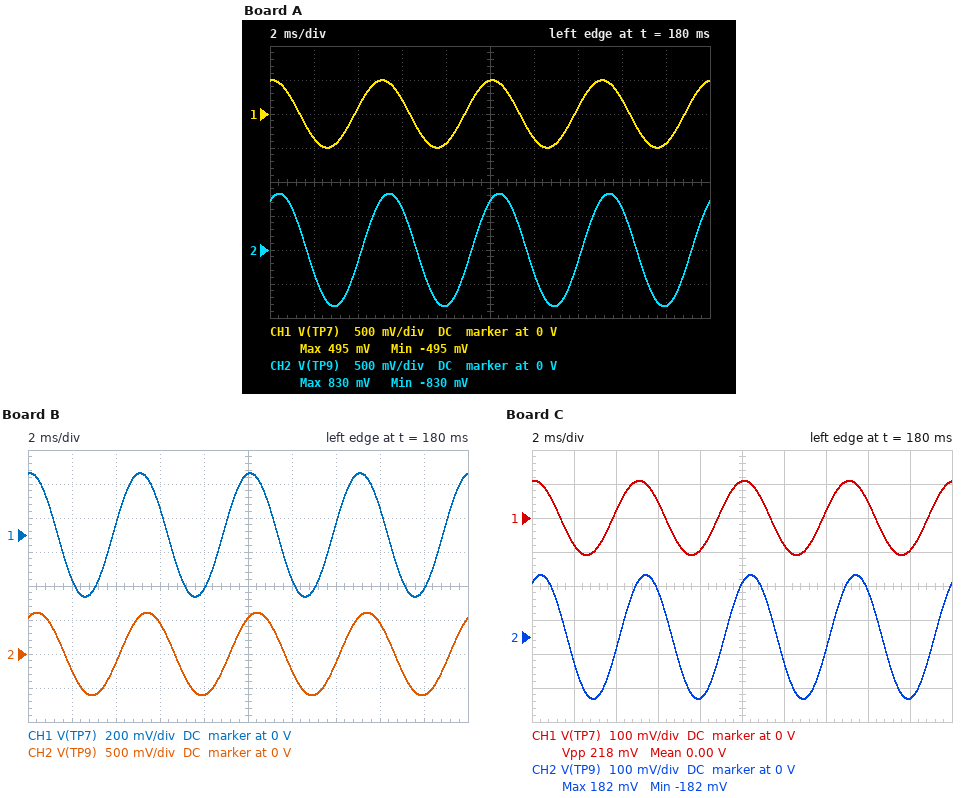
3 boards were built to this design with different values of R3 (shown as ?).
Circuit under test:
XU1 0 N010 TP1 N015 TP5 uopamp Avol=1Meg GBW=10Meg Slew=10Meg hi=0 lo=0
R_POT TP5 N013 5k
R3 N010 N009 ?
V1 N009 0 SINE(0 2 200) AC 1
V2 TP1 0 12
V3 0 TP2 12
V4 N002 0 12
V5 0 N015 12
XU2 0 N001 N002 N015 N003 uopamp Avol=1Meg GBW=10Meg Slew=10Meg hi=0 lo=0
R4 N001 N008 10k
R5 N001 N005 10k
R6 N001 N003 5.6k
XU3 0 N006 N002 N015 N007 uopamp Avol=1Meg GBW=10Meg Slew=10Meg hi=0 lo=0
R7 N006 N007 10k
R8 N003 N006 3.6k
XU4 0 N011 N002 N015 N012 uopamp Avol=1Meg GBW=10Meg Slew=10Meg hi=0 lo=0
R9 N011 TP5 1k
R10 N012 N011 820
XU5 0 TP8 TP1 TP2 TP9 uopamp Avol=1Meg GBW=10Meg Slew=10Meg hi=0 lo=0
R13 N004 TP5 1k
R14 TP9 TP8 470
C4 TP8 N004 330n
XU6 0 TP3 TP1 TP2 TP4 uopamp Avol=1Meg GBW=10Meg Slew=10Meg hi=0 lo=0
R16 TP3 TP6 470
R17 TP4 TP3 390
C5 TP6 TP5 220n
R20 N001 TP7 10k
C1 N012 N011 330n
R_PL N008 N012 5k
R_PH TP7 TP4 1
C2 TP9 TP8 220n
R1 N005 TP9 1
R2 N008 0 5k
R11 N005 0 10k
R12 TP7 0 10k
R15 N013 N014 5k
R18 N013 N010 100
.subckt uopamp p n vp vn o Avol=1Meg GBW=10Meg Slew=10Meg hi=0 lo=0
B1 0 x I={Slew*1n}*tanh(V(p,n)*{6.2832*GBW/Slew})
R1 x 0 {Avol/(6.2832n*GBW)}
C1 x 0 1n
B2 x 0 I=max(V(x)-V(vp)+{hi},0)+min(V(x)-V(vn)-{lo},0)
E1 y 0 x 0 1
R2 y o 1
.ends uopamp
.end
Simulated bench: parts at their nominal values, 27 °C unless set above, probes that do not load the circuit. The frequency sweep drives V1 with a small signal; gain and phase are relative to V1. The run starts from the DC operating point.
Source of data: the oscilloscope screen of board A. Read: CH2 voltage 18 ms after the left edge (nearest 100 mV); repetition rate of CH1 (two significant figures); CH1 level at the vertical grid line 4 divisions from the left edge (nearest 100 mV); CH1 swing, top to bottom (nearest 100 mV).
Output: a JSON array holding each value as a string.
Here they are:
["-800 mV", "200 Hz", "-400 mV", "1.0 V"]
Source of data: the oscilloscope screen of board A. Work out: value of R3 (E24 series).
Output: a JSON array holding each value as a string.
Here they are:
["2.2 kΩ"]
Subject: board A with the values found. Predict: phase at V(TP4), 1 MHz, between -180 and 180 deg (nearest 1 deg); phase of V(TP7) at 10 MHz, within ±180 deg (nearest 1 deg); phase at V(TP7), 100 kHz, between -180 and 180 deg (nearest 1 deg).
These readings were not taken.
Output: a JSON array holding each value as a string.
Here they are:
["-29 deg", "-135 deg", "-2 deg"]
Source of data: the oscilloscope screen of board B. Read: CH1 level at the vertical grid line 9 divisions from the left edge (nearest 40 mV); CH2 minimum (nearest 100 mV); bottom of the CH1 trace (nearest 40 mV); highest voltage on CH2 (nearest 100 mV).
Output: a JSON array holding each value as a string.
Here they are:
["-320 mV", "-600 mV", "-360 mV", "600 mV"]
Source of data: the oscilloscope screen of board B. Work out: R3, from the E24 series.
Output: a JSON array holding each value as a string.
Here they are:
["3 kΩ"]
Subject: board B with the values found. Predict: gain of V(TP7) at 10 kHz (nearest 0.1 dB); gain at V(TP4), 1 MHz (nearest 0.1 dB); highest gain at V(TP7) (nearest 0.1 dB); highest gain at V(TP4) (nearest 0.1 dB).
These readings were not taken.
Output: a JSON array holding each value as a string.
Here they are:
["2.9 dB", "2.5 dB", "3.0 dB", "3.0 dB"]
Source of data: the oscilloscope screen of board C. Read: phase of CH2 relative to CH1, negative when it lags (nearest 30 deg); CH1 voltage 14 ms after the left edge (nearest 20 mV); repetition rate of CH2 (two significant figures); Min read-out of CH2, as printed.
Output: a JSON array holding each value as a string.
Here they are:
["-30 deg", "20 mV", "200 Hz", "-182 mV"]
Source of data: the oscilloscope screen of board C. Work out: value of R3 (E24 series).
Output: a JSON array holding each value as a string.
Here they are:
["10 kΩ"]
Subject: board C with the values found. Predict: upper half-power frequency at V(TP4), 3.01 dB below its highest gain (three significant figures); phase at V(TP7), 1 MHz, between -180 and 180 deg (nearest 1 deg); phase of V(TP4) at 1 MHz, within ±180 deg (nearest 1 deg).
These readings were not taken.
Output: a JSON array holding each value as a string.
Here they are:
["3.84 MHz", "-19 deg", "-19 deg"]
